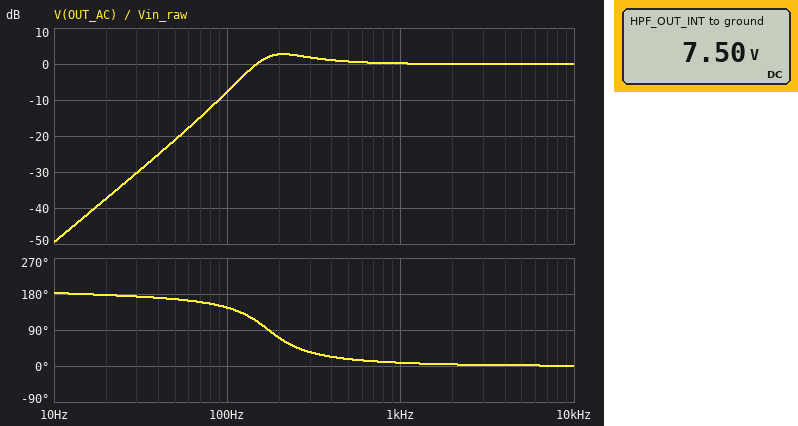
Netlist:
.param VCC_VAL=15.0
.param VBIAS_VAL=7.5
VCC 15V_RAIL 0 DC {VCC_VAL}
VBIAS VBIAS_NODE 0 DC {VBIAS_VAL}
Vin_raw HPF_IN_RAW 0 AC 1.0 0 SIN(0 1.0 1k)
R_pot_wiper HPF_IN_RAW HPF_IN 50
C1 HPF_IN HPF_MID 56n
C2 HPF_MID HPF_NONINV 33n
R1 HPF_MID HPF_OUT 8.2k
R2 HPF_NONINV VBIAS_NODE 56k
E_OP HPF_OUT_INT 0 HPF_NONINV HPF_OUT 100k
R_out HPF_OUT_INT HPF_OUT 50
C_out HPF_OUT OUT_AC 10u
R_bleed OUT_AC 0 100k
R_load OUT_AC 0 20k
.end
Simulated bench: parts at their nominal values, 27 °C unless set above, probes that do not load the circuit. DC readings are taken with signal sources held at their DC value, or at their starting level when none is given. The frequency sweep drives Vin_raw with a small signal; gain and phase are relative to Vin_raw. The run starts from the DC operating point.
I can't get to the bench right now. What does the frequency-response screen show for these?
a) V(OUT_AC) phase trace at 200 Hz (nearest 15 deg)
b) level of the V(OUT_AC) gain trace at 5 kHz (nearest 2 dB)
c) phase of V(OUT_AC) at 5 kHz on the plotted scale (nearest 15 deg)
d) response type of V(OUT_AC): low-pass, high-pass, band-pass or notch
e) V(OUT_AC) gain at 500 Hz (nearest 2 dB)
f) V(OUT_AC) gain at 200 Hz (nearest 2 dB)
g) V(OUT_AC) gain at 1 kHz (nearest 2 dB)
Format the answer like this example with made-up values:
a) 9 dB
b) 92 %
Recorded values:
a) 75 deg
b) 0 dB
c) 0 deg
d) high-pass
e) 0 dB
f) 2 dB
g) 0 dB
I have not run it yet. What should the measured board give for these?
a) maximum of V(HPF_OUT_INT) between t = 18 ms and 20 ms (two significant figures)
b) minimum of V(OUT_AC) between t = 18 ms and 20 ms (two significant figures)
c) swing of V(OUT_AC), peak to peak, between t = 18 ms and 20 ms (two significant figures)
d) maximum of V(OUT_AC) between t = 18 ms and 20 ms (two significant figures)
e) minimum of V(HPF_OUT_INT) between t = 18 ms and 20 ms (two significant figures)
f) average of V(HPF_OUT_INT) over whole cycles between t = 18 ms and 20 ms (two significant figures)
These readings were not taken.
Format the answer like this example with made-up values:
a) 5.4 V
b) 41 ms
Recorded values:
a) 8.5 V
b) -1.0 V
c) 2.0 V
d) 1.0 V
e) 6.5 V
f) 7.5 V
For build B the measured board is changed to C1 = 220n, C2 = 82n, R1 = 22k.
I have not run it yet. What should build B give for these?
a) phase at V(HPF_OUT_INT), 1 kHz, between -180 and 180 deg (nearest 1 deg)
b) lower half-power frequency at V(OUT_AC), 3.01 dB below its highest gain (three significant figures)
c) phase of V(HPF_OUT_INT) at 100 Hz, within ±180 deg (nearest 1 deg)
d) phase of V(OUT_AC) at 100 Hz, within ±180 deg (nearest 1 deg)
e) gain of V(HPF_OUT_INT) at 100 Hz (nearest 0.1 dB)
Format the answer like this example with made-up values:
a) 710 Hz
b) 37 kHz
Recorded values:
a) 3 deg
b) 33.7 Hz
c) 28 deg
d) 29 deg
e) 0 dB
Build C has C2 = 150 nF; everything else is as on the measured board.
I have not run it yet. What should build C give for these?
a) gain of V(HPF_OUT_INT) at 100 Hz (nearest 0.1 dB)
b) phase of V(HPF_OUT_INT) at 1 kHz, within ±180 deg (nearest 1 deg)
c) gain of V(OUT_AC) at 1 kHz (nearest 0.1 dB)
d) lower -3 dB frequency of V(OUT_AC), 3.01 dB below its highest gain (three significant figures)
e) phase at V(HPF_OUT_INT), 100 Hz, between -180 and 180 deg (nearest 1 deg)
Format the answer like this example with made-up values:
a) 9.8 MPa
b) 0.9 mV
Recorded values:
a) 2.2 dB
b) 4 deg
c) 0 dB
d) 68.3 Hz
e) 64 deg
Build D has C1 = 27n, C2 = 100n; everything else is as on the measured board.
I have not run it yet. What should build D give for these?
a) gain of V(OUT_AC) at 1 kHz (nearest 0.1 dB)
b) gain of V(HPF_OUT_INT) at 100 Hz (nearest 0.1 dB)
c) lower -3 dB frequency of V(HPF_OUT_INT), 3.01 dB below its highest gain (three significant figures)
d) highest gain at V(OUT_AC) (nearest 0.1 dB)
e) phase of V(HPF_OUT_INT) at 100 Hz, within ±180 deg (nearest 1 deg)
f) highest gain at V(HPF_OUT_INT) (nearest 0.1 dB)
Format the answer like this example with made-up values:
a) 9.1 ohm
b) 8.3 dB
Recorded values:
a) 0.1 dB
b) -4.6 dB
c) 121 Hz
d) 1.6 dB
e) 128 deg
f) 1.7 dB
